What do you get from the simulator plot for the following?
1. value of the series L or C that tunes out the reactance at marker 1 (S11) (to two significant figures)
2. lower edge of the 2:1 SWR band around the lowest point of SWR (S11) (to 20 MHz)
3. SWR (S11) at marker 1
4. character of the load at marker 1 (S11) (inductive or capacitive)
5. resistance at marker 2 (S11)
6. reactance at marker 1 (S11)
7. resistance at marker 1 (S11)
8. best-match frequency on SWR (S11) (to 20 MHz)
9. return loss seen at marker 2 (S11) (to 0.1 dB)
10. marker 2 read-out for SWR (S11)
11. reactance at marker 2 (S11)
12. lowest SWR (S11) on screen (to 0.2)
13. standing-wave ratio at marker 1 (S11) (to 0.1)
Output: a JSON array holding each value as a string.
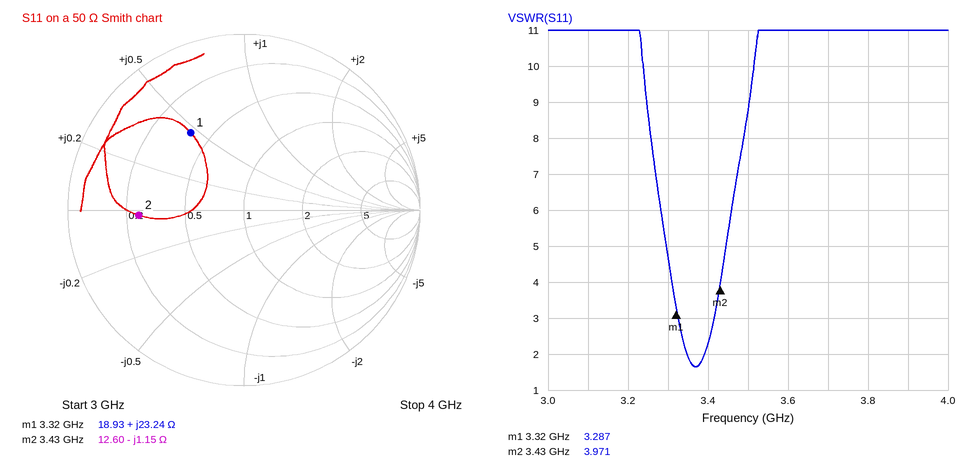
["2.1 pF", "3.34 GHz", "3.287", "inductive", "12.60 Ω", "+23.24 Ω", "18.93 Ω", "3.36 GHz", "4.5 dB", "3.971", "-1.15 Ω", "1.6", "3.3"]
